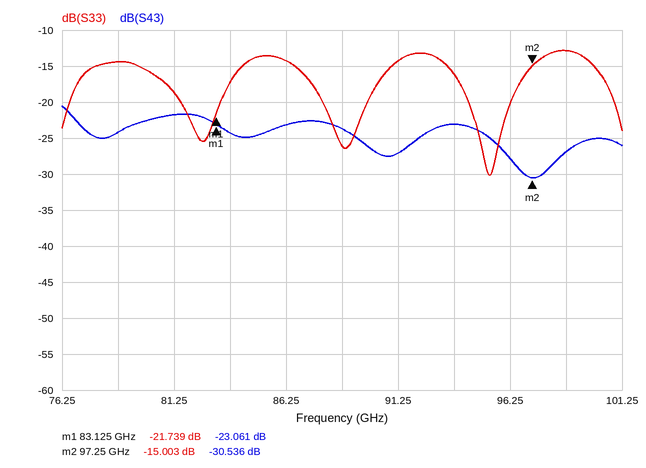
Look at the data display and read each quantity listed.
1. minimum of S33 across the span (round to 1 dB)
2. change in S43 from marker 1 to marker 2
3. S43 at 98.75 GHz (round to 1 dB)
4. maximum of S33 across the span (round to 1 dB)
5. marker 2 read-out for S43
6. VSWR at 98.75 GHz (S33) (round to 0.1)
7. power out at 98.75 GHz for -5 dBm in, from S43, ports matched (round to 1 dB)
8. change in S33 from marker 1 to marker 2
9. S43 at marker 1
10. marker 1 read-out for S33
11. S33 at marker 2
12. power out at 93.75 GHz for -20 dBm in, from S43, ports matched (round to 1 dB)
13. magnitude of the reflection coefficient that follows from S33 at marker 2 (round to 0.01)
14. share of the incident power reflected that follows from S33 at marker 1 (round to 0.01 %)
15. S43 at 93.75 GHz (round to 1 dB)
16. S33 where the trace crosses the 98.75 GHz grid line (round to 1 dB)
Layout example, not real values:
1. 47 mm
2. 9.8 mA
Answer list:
1. -30 dB
2. -7.475 dB
3. -27 dB
4. -13 dB
5. -30.536 dB
6. 1.6
7. -32 dBm
8. 6.736 dB
9. -23.061 dB
10. -21.739 dB
11. -15.003 dB
12. -43 dBm
13. 0.18
14. 0.67 %
15. -23 dB
16. -13 dB
